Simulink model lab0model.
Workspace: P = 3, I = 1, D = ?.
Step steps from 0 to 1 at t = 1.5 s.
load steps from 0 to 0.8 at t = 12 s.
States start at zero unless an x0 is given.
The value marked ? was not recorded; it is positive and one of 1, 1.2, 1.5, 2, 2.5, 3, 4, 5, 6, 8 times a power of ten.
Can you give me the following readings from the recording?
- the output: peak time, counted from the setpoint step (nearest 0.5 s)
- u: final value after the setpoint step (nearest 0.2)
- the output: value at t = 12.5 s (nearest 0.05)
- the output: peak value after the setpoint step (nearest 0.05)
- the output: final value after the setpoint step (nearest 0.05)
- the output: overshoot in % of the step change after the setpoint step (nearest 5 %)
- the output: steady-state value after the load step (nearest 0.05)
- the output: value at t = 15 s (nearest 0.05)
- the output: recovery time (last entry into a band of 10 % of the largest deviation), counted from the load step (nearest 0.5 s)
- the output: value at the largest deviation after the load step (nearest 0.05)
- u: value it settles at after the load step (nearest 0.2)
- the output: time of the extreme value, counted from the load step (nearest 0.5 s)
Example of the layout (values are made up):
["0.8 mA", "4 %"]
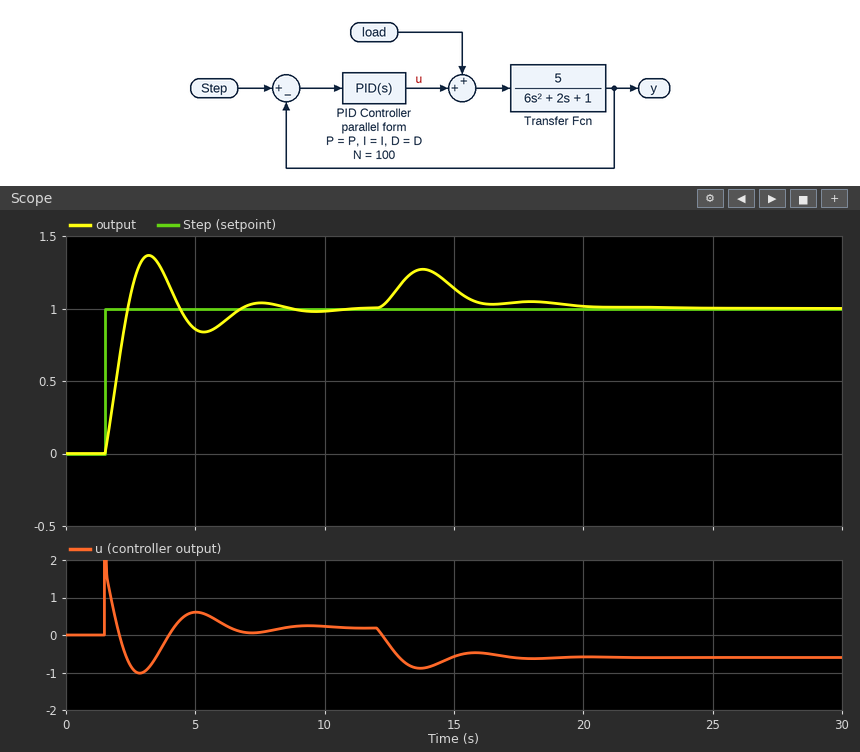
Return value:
["1.5 s", "0.2", "1.05", "1.35", "1.00", "35 %", "1.00", "1.15", "7.5 s", "1.25", "-0.6", "2.0 s"]
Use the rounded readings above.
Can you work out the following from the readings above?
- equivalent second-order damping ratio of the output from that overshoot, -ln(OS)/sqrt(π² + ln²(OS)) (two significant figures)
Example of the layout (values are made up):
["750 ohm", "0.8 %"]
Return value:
["0.32"]
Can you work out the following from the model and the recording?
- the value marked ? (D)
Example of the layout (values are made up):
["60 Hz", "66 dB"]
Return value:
["1.2"]
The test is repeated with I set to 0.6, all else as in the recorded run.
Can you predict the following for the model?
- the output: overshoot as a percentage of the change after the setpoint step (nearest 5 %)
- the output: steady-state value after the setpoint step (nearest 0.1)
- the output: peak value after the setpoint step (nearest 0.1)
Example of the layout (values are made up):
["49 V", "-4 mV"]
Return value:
["30 %", "1.0", "1.3"]
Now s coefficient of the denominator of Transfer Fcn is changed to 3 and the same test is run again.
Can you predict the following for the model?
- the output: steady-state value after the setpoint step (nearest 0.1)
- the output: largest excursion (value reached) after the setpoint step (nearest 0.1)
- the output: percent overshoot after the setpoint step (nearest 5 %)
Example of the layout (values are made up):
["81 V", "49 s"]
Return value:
["1.0", "1.3", "30 %"]
